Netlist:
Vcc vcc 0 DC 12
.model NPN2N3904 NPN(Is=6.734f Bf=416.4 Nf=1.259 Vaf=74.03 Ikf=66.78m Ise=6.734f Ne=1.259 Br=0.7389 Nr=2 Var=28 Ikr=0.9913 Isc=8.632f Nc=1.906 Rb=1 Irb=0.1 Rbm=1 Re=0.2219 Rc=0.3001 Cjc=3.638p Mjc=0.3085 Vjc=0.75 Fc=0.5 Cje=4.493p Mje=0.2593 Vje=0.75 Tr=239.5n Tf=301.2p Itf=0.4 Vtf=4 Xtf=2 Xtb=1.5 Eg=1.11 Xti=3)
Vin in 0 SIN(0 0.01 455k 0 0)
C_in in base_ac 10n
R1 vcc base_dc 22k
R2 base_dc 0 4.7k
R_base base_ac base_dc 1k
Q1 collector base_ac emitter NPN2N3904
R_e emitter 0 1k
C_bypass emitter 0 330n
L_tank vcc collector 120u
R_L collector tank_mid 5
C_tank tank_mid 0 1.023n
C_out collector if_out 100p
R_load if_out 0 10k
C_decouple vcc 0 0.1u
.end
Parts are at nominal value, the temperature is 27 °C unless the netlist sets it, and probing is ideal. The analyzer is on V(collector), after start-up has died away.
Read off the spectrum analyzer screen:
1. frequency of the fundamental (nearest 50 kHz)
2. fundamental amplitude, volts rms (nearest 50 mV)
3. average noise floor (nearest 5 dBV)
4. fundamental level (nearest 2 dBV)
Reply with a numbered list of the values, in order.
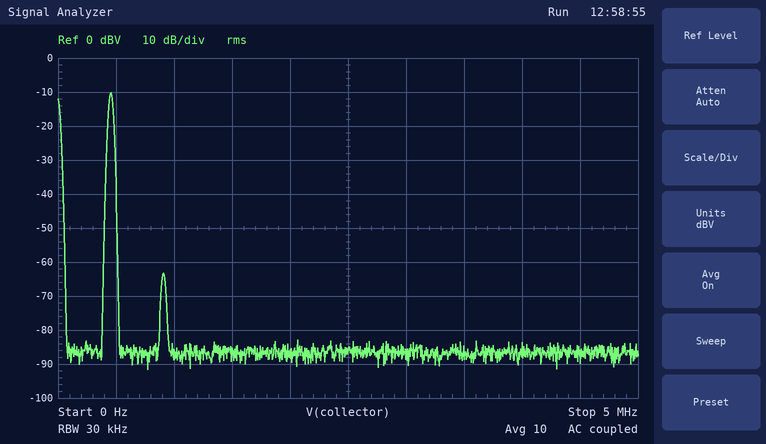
1. 450 kHz
2. 300 mV
3. -85 dBV
4. -10 dBV
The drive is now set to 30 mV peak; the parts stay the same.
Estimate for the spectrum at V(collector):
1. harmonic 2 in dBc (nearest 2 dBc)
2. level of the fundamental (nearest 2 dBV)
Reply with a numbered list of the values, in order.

1. -44 dBc
2. -2 dBV
